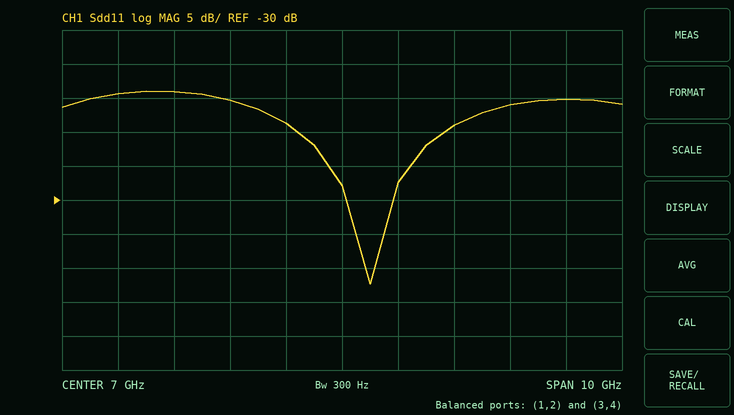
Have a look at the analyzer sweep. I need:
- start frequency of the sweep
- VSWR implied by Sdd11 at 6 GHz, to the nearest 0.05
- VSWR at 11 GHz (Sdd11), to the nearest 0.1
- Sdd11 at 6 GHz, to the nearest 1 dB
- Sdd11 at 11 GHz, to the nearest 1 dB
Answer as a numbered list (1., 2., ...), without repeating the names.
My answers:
1. 2 GHz
2. 1.25
3. 1.4
4. -19 dB
5. -15 dB
